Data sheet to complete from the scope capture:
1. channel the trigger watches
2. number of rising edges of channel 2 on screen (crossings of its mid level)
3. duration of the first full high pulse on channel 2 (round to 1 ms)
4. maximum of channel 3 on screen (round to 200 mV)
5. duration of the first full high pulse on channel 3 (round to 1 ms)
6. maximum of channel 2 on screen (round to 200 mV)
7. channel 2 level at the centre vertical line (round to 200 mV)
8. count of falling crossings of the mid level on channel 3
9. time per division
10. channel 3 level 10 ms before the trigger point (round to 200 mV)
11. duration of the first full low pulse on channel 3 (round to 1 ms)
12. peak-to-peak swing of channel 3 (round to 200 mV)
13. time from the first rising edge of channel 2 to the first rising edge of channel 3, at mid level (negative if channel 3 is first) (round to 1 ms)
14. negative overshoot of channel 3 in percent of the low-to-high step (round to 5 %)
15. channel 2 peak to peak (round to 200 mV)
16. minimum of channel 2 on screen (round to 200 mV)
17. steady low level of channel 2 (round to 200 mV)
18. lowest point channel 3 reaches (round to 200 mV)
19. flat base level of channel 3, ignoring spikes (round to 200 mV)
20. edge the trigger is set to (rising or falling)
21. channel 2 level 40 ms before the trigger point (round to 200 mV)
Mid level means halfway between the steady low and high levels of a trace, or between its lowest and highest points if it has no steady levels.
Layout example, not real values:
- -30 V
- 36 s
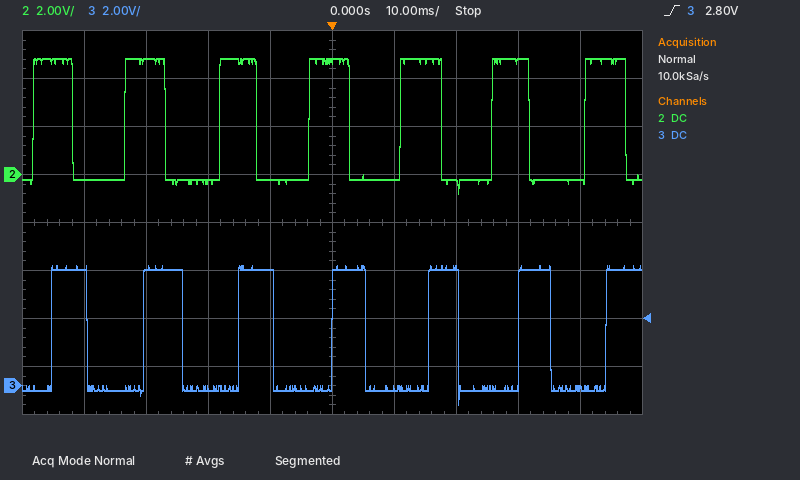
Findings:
- channel 3
- 7
- 6 ms
- 5.0 V
- 6 ms
- 4.8 V
- 4.8 V
- 6
- 10 ms
- 4.8 V
- 9 ms
- 5.8 V
- +3 ms
- 10 %
- 5.6 V
- -800 mV
- -200 mV
- -800 mV
- -200 mV
- rising
- -200 mV
